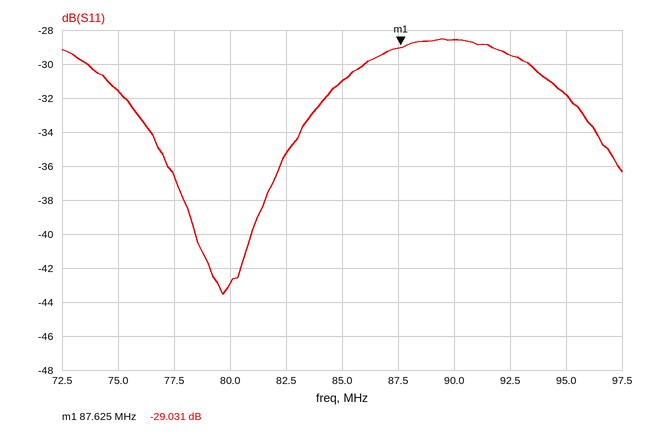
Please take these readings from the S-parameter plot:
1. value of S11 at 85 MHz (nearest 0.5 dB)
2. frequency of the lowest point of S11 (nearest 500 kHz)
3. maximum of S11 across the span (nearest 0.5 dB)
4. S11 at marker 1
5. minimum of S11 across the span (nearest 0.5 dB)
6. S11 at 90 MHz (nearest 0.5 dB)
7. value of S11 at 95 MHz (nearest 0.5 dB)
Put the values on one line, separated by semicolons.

-31.0 dB; 79.5 MHz; -28.5 dB; -29.031 dB; -43.5 dB; -28.5 dB; -32.0 dB
